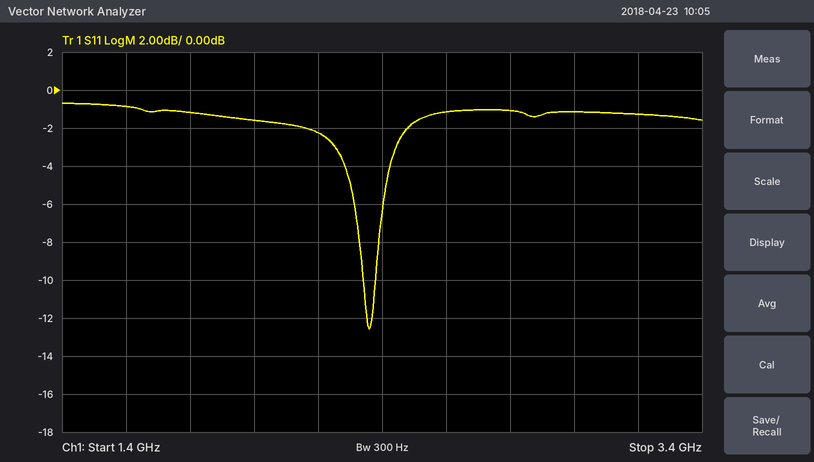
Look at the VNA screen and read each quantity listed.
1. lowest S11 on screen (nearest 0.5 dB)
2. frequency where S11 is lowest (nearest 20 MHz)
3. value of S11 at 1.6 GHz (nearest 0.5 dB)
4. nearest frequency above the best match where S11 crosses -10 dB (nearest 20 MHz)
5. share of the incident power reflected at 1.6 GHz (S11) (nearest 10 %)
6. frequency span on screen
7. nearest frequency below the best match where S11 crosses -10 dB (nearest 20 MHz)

-12.5 dB
2.36 GHz
-1.0 dB
2.38 GHz
80 %
2 GHz
2.34 GHz
